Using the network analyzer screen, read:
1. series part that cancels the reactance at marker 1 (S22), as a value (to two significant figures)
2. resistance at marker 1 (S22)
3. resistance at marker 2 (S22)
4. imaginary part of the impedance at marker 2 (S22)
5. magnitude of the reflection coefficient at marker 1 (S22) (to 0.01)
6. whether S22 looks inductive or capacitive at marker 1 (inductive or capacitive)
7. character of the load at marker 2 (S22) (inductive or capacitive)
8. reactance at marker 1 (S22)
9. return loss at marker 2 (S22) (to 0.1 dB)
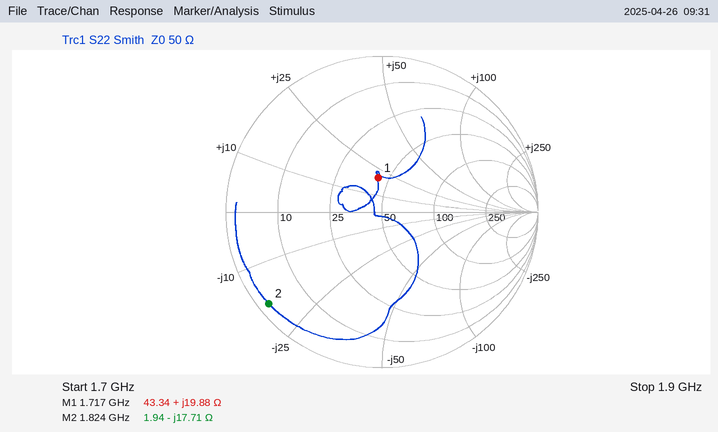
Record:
4.7 pF
43.34 Ω
1.94 Ω
-17.71 Ω
0.22
inductive
capacitive
+19.88 Ω
0.6 dB
